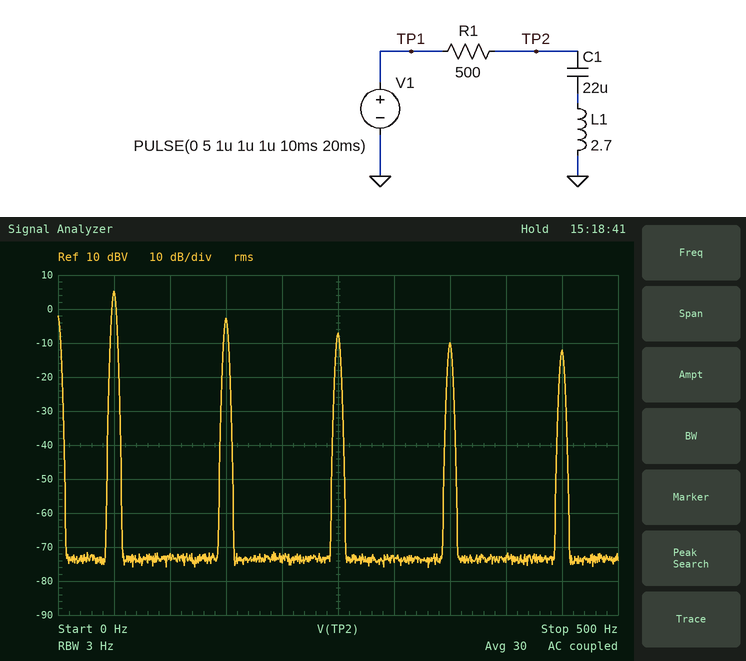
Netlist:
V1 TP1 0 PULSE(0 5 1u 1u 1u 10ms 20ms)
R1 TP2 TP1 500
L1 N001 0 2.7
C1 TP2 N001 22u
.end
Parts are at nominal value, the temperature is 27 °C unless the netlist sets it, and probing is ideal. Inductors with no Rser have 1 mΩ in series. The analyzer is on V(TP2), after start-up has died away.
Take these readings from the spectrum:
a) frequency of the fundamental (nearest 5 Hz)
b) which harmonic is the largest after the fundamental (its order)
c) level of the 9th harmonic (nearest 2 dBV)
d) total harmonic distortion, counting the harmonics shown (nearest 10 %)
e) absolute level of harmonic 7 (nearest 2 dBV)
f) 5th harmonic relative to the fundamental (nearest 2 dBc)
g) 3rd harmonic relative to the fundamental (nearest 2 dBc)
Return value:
50 Hz
3
-12 dBV
50 %
-10 dBV
-12 dBc
-8 dBc
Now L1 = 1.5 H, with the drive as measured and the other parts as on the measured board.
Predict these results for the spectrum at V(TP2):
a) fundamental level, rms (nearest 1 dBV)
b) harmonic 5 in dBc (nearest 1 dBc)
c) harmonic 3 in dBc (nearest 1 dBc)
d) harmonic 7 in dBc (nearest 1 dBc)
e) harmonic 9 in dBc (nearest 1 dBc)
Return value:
2 dBV
-9 dBc
-5 dBc
-12 dBc
-14 dBc
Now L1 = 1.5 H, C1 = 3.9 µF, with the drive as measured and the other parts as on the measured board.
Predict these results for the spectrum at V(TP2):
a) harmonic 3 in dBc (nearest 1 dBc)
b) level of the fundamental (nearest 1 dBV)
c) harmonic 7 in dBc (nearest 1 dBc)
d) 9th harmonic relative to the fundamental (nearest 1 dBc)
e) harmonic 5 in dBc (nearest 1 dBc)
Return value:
-5 dBc
2 dBV
-12 dBc
-14 dBc
-9 dBc
